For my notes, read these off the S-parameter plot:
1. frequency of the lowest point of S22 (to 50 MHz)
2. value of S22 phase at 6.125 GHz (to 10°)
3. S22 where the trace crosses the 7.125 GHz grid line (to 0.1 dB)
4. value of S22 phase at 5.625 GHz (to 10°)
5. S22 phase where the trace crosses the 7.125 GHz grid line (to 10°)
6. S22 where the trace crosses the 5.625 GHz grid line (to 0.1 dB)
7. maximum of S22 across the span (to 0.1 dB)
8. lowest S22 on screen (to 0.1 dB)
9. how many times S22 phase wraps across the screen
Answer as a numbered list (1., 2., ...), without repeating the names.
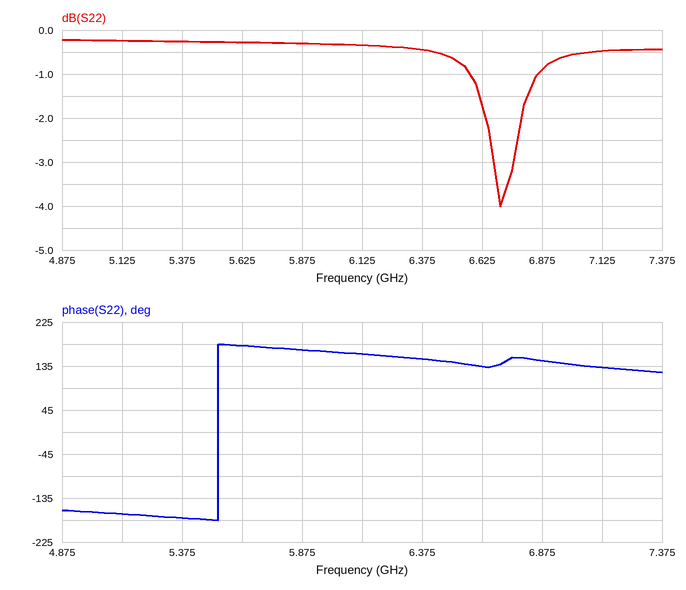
1. 6.70 GHz
2. 160°
3. -0.5 dB
4. 180°
5. 130°
6. -0.3 dB
7. -0.2 dB
8. -4.0 dB
9. 1
